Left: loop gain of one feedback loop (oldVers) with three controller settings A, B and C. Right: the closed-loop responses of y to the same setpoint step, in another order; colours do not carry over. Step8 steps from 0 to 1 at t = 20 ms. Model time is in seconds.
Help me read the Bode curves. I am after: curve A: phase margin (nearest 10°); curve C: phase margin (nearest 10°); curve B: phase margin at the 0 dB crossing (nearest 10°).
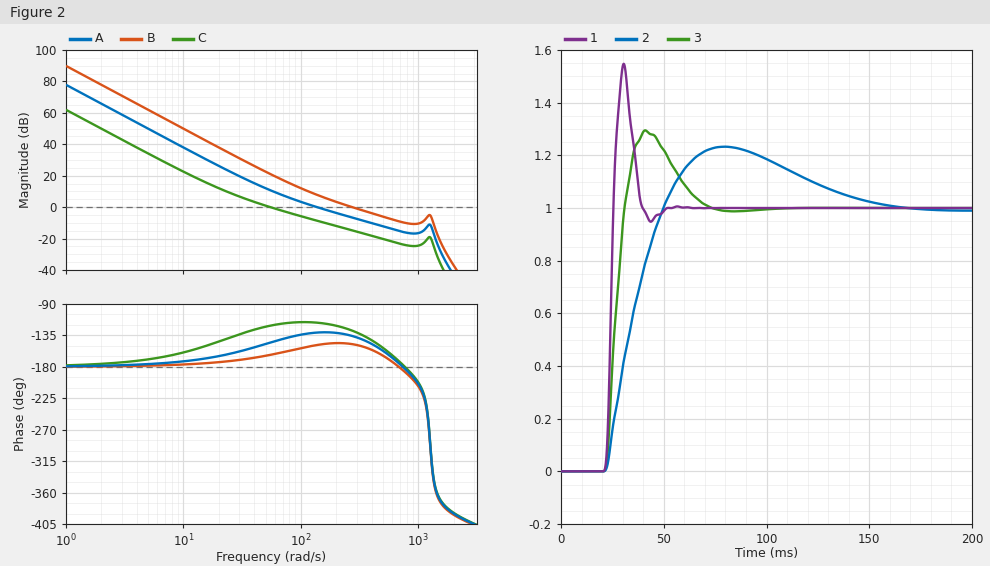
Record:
50°
60°
30°
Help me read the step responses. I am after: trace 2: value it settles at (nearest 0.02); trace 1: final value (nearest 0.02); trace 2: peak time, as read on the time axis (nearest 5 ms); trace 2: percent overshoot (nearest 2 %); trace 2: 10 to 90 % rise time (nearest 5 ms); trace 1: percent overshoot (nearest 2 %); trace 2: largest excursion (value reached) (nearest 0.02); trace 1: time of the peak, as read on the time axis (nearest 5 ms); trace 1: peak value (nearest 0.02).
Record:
1.00
1.00
80 ms
24 %
20 ms
54 %
1.24
30 ms
1.54
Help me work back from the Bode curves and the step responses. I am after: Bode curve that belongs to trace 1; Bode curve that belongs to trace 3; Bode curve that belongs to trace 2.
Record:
B
A
C
